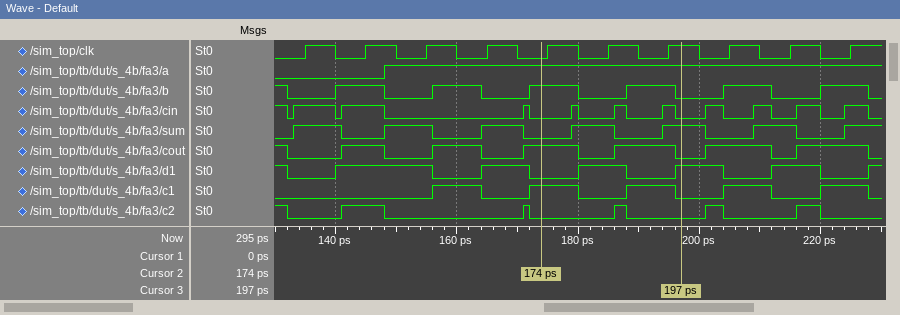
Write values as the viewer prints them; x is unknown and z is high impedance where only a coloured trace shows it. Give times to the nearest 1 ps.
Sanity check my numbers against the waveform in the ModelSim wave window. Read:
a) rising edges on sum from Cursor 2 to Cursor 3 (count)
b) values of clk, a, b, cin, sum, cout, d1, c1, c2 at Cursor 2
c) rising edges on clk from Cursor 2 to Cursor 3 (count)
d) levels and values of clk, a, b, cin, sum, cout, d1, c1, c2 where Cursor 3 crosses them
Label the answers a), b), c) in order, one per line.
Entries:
a) 2
b) clk=0, a=1, b=1, cin=0, sum=0, cout=1, d1=0, c1=1, c2=0
c) 3
d) clk=1, a=1, b=0, cin=0, sum=1, cout=0, d1=1, c1=0, c2=0
